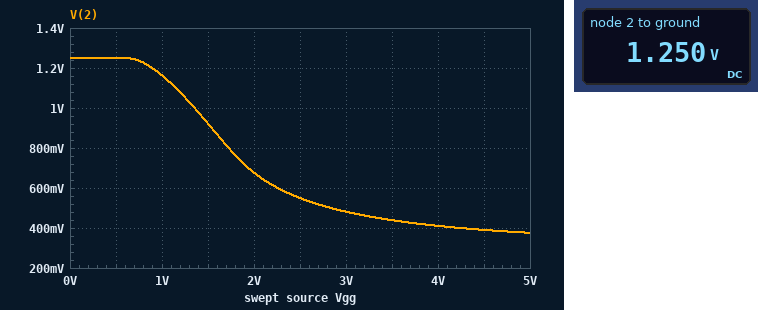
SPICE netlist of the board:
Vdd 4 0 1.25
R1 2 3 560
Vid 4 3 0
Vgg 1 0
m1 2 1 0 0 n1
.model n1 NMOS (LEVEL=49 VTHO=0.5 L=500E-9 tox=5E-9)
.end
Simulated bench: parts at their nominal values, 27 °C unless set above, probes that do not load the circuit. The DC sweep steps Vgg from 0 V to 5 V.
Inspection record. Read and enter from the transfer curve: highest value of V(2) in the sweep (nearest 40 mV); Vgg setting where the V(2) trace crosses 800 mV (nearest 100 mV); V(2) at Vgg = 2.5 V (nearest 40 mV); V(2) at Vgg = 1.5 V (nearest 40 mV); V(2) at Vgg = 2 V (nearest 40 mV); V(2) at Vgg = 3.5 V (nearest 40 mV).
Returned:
1.24 V
1.7 V
560 mV
920 mV
680 mV
440 mV
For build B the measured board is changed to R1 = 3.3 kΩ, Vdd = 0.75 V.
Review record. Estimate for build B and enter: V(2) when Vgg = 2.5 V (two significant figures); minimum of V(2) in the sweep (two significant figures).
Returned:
67 mV
46 mV
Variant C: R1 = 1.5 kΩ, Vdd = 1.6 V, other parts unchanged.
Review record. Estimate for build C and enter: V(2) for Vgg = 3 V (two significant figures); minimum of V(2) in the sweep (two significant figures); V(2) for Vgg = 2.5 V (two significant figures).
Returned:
280 mV
210 mV
320 mV
